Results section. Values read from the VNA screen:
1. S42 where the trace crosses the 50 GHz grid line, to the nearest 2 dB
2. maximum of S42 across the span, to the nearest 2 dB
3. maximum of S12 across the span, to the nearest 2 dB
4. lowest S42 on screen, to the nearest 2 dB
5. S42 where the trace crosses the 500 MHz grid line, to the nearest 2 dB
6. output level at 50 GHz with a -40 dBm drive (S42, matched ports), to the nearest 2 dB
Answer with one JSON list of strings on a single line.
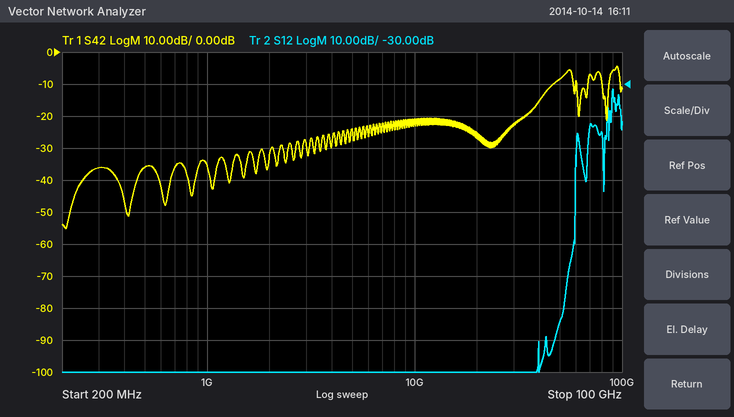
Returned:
["-8 dB", "-4 dB", "-32 dB", "-56 dB", "-36 dB", "-48 dBm"]
